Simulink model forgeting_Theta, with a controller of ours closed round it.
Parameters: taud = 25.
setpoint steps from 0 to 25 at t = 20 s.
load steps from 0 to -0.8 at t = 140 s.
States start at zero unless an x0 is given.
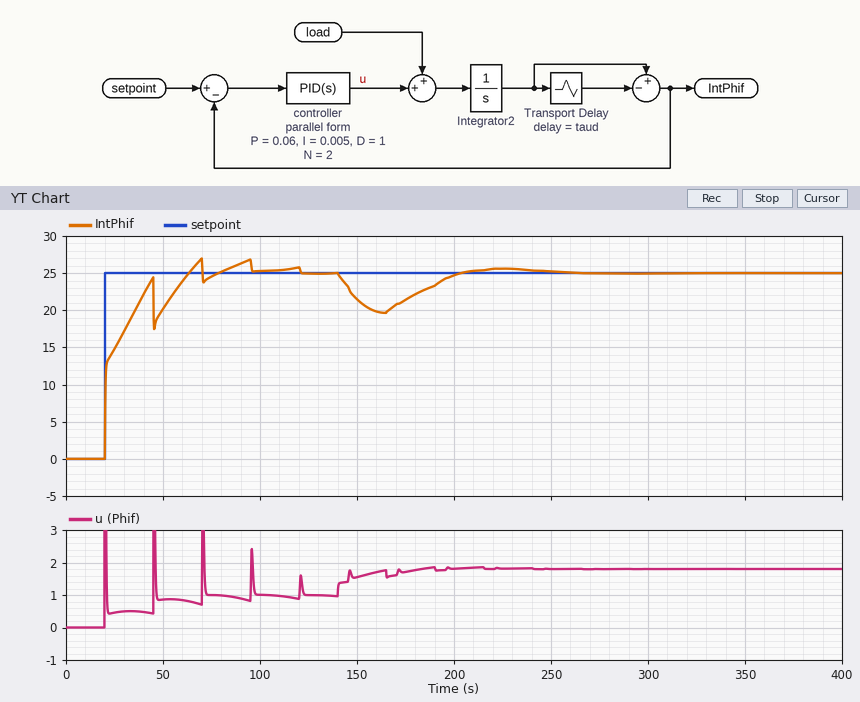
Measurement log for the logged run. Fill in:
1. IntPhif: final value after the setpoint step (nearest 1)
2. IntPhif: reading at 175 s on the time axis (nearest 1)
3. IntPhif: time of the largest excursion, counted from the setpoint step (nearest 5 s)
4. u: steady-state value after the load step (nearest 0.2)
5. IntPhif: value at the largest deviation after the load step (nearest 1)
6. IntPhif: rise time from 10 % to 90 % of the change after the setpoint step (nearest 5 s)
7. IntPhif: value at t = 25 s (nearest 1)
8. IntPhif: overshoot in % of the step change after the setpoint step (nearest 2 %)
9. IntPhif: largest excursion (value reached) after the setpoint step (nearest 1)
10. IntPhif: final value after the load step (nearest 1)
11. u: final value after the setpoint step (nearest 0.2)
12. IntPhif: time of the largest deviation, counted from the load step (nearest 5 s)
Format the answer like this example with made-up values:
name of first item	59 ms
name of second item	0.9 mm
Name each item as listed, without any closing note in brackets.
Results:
IntPhif: final value after the setpoint step	25
IntPhif: reading at 175 s on the time axis	21
IntPhif: time of the largest excursion, counted from the setpoint step	50 s
u: steady-state value after the load step	1.8
IntPhif: value at the largest deviation after the load step	20
IntPhif: rise time from 10 % to 90 % of the change after the setpoint step	20 s
IntPhif: value at t = 25 s	15
IntPhif: overshoot in % of the step change after the setpoint step	8 %
IntPhif: largest excursion (value reached) after the setpoint step	27
IntPhif: final value after the load step	25
u: final value after the setpoint step	1.0
IntPhif: time of the largest deviation, counted from the load step	25 s
